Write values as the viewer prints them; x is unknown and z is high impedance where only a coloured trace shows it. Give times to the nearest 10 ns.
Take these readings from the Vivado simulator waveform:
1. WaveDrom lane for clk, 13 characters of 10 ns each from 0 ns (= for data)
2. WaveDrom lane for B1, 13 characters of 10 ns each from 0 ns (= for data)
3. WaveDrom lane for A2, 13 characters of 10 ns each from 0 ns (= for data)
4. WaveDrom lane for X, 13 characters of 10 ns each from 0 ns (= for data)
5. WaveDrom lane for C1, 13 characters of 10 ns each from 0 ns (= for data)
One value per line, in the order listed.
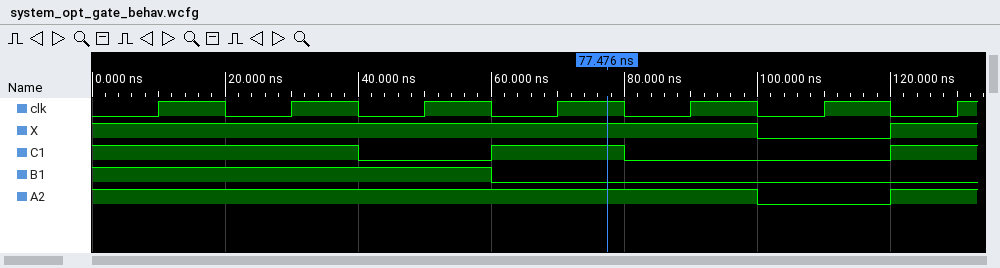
{name: 'clk', wave: '0101010101010'}
{name: 'B1', wave: '1.....0......'}
{name: 'A2', wave: '1.........0.1'}
{name: 'X', wave: '1.........0.1'}
{name: 'C1', wave: '1...0.1.0...1'}
